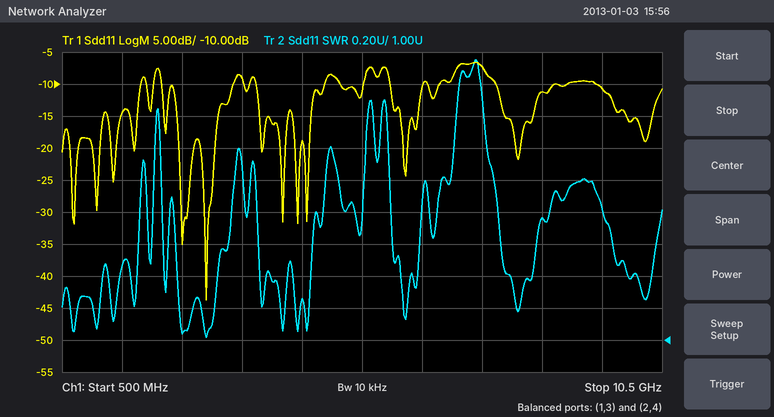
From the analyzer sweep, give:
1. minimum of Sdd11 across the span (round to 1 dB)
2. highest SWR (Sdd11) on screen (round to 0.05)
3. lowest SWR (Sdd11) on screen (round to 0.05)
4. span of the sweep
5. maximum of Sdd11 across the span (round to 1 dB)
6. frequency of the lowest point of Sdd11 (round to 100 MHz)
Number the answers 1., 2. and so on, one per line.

1. -44 dB
2. 2.75
3. 1.00
4. 10 GHz
5. -7 dB
6. 2.9 GHz
